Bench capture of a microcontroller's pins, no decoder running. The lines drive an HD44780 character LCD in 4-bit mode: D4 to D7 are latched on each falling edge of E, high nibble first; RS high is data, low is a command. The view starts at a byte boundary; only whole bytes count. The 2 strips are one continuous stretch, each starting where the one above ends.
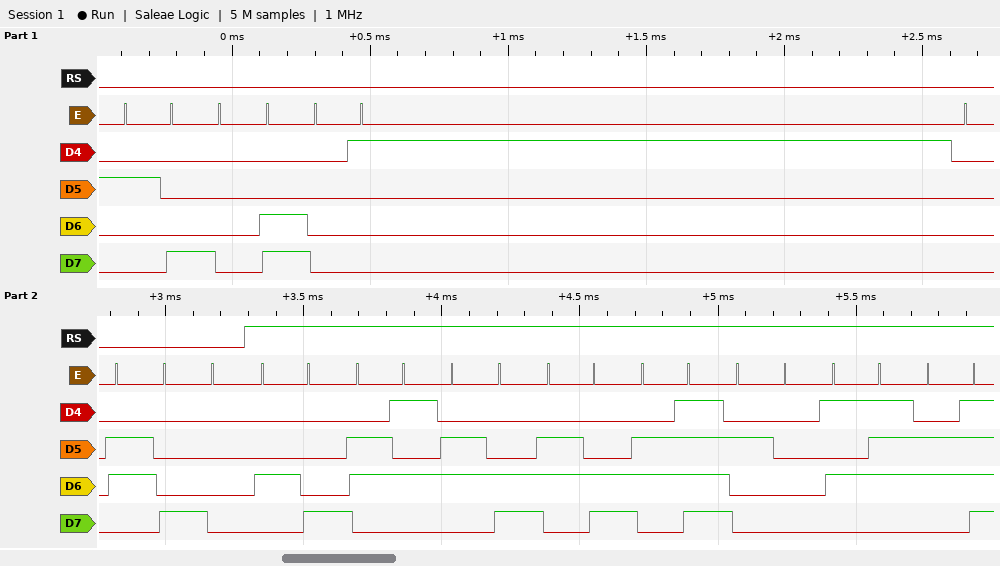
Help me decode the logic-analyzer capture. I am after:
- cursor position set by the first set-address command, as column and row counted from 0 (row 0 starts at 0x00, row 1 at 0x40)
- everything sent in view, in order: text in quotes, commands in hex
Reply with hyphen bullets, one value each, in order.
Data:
- column 0, row 0
- 0x28 0x0C 0x01 0x06 0x80 "Hello Wo"
